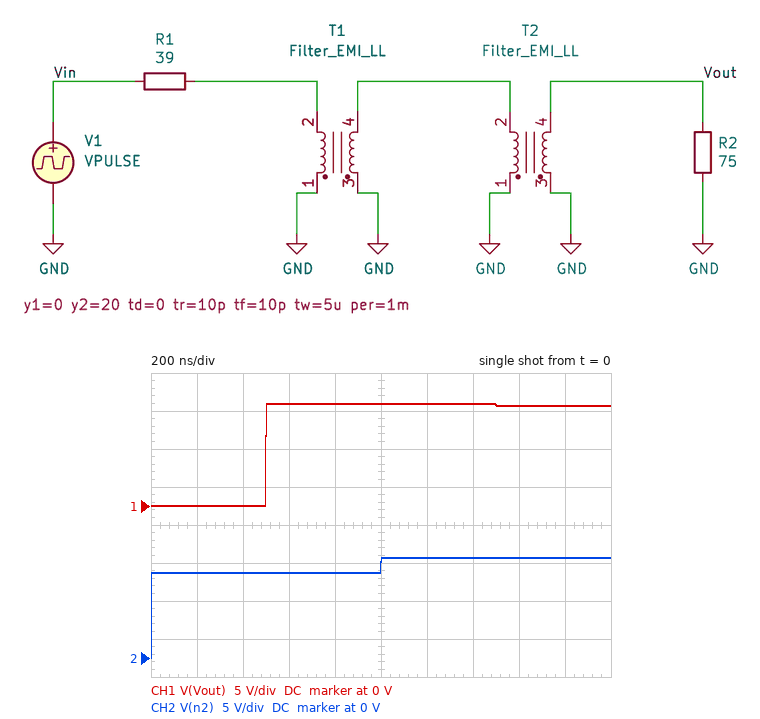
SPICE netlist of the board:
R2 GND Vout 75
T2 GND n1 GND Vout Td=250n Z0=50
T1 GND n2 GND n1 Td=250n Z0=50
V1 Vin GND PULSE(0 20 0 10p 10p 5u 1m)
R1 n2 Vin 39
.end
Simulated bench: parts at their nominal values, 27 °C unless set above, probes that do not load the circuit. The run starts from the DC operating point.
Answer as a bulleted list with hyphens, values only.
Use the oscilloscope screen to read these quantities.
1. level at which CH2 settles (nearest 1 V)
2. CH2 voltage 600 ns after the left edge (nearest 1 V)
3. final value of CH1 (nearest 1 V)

- 13 V
- 11 V
- 13 V
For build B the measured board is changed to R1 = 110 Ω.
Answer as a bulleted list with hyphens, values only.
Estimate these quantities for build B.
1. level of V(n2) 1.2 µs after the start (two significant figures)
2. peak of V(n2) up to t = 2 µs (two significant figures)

- 8.0 V
- 8.1 V
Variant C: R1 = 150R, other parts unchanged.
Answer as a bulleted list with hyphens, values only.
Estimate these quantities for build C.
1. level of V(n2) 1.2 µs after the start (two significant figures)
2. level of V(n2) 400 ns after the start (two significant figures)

- 6.5 V
- 5.0 V
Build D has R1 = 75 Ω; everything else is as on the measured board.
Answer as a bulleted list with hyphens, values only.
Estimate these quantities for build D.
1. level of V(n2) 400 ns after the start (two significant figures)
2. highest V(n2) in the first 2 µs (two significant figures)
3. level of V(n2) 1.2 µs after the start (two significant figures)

- 8.0 V
- 10 V
- 9.9 V
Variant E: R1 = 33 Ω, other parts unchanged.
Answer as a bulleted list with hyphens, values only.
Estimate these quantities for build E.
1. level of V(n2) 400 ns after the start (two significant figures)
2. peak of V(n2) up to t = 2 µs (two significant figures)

- 12 V
- 14 V
